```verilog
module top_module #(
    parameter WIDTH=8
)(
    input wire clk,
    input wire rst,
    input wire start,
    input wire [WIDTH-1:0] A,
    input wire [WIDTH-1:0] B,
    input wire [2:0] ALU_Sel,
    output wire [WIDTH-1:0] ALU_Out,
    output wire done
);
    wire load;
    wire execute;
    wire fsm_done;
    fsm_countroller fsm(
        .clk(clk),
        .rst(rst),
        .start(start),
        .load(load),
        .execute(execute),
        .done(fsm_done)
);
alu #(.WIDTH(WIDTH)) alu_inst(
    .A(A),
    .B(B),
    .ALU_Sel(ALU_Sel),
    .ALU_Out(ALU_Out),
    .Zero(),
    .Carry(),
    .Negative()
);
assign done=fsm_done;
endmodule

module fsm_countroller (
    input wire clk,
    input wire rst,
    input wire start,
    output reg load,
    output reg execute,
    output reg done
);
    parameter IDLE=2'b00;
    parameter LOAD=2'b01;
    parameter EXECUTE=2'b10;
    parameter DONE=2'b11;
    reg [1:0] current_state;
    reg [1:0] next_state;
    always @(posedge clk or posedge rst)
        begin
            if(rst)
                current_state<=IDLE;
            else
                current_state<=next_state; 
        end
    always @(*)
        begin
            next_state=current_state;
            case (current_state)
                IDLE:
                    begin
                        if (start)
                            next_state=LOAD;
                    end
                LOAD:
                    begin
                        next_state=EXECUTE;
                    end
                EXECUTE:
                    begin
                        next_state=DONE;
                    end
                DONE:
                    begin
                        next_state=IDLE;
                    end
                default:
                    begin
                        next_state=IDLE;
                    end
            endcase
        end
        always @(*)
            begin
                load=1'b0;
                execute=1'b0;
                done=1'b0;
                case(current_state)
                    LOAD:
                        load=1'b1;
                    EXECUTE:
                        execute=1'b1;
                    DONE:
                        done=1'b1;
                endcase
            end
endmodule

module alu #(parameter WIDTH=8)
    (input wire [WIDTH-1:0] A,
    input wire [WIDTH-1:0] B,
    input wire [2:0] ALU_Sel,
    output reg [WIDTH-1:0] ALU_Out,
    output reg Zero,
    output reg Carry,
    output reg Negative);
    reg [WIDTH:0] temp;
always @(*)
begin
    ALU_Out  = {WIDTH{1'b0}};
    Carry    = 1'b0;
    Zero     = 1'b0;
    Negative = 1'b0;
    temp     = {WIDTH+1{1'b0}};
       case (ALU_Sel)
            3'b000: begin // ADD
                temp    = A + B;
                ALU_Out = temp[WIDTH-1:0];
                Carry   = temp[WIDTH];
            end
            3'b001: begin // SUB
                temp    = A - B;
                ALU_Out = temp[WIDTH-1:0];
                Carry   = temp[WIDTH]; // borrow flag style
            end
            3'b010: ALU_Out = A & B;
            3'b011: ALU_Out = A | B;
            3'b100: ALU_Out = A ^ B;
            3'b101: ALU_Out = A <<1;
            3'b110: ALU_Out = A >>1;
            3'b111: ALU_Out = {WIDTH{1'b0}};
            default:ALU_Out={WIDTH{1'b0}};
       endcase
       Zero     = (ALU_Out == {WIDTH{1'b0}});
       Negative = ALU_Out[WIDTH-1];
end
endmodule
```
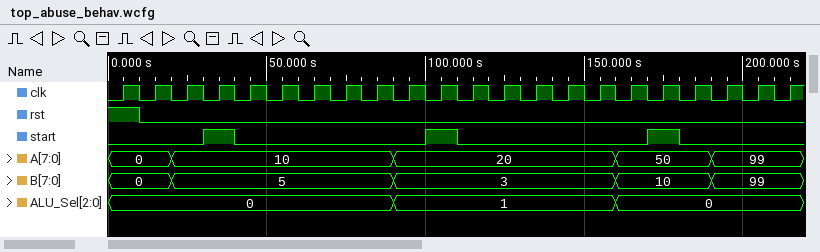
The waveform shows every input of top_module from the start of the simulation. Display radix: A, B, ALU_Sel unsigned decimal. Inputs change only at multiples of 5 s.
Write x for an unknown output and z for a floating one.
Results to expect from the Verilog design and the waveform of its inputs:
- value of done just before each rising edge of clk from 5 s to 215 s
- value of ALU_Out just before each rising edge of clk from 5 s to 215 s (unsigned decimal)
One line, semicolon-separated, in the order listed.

0 0 0 0 0 0 1 0 0 0 0 0 0 1 0 0 0 0 0 0 1 0; 0, 0, 15, 15, 15, 15, 15, 15, 15, 17, 17, 17, 17, 17, 17, 17, 60, 60, 60, 198, 198, 198
